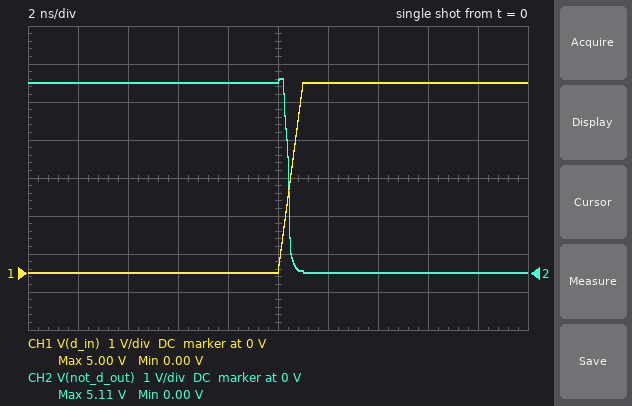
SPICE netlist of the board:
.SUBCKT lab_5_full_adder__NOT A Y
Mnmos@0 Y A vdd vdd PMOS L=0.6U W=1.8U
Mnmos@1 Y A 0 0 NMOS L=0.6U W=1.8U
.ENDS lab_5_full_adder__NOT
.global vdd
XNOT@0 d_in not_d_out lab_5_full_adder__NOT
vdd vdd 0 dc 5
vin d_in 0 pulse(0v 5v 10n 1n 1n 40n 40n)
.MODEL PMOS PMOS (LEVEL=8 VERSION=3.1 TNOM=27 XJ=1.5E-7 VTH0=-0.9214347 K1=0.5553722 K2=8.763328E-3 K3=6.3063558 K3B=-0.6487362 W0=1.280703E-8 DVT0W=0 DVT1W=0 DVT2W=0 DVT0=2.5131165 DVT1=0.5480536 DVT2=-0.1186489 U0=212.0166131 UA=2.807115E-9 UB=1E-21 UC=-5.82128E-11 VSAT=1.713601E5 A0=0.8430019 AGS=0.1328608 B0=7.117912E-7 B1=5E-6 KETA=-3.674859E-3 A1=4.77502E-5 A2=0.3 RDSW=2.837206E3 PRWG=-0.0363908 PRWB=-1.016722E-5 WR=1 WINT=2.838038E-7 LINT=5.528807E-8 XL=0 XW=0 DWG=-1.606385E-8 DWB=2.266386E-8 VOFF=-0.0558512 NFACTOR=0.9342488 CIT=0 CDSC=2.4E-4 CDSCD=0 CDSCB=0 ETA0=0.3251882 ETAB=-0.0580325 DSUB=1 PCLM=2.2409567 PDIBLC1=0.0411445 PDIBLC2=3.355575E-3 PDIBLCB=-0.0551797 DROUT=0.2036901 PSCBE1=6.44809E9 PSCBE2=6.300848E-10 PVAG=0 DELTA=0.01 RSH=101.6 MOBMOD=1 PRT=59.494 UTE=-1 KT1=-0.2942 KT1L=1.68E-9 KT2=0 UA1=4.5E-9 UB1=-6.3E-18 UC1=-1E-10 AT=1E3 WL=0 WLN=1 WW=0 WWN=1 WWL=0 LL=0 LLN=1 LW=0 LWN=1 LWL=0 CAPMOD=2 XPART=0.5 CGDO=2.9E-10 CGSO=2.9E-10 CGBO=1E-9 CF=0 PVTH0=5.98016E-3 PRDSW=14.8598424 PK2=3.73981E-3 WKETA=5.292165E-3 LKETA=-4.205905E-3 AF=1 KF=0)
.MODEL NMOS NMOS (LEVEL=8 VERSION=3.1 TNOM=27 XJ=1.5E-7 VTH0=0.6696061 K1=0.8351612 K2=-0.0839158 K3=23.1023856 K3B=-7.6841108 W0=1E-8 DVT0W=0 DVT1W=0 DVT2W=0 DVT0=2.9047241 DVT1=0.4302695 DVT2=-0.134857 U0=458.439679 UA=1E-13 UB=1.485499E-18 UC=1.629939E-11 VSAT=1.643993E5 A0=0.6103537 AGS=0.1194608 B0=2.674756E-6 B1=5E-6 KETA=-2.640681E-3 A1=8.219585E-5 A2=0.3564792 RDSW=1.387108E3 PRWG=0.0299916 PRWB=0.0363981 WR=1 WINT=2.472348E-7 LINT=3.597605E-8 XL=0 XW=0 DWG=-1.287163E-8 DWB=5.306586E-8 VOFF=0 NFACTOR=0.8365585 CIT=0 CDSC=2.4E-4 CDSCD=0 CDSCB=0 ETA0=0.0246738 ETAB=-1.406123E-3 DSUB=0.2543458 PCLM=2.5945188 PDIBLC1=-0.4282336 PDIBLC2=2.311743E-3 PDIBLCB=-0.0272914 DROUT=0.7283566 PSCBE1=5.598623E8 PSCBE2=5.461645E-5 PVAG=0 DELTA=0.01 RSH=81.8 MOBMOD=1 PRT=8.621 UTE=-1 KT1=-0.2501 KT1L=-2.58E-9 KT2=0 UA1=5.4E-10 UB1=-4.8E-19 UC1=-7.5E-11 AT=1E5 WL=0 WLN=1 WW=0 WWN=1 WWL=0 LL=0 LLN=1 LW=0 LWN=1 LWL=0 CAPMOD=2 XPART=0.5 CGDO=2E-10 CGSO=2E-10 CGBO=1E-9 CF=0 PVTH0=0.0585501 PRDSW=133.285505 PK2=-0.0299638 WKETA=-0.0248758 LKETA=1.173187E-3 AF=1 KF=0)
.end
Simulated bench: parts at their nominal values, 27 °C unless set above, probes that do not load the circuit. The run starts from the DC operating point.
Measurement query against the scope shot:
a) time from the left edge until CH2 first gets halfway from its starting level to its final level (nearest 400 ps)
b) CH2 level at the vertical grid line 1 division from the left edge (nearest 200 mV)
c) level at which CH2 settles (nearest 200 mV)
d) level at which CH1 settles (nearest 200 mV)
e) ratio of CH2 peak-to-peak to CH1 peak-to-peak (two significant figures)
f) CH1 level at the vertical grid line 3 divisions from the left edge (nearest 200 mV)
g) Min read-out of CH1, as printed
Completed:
10.4 ns
5.0 V
0 V
5.0 V
1.0
0 V
0.00 V
